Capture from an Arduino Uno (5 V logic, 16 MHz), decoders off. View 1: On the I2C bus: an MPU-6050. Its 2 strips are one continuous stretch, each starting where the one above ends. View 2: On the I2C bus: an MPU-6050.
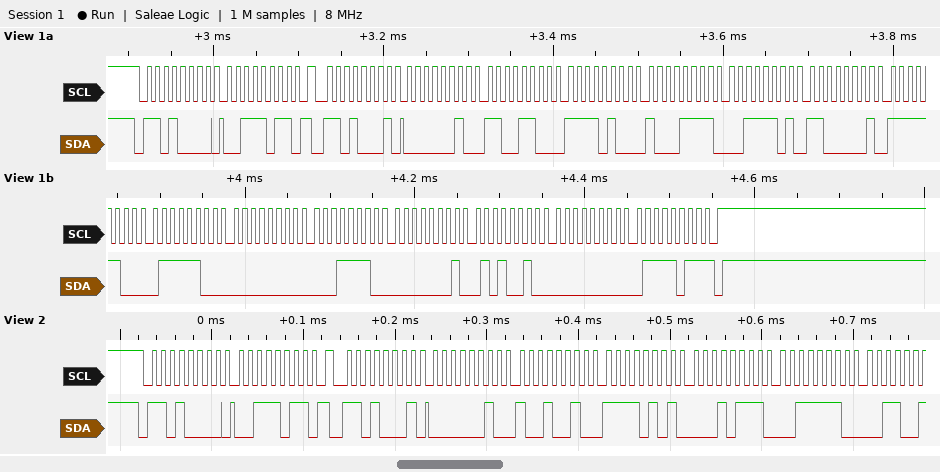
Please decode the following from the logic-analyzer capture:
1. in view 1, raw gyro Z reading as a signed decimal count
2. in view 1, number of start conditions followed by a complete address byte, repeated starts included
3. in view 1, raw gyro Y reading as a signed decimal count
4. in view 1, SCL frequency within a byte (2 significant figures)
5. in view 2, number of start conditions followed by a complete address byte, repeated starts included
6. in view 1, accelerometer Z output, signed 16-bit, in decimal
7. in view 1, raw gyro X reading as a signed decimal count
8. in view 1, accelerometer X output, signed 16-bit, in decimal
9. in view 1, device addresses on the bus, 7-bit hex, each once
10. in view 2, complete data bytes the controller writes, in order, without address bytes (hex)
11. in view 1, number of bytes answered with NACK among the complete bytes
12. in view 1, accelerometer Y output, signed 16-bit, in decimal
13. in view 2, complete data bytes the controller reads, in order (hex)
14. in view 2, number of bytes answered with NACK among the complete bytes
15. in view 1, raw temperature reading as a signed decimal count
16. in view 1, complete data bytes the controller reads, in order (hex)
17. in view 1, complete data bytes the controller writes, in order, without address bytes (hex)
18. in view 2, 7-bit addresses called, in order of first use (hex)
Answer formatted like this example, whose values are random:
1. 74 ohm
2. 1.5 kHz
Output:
1. 123
2. 2
3. 338
4. 100 kHz
5. 2
6. 15809
7. 30
8. 716
9. 0x68
10. 3B
11. 1
12. -2929
13. 02 92 F5 17 3E
14. 0
15. -900
16. 02 CC F4 8F 3D C1 FC 7C 00 1E 01 52 00 7B
17. 3B
18. 0x68
